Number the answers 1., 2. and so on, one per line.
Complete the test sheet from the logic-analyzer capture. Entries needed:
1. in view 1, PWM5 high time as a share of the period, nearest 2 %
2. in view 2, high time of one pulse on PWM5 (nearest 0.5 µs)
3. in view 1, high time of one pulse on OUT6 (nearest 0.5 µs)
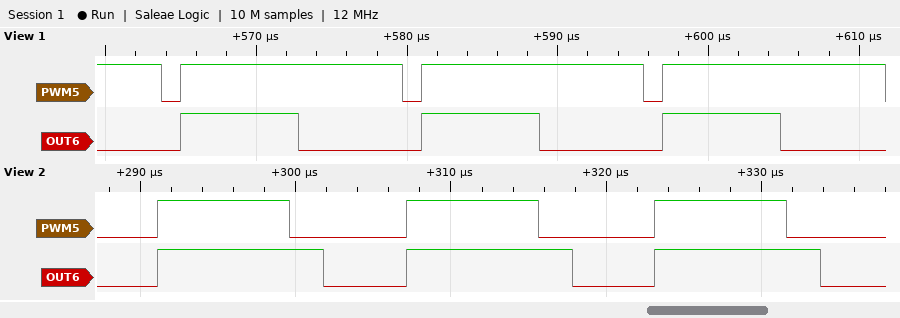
1. 92 %
2. 8.5 µs
3. 8.0 µs
